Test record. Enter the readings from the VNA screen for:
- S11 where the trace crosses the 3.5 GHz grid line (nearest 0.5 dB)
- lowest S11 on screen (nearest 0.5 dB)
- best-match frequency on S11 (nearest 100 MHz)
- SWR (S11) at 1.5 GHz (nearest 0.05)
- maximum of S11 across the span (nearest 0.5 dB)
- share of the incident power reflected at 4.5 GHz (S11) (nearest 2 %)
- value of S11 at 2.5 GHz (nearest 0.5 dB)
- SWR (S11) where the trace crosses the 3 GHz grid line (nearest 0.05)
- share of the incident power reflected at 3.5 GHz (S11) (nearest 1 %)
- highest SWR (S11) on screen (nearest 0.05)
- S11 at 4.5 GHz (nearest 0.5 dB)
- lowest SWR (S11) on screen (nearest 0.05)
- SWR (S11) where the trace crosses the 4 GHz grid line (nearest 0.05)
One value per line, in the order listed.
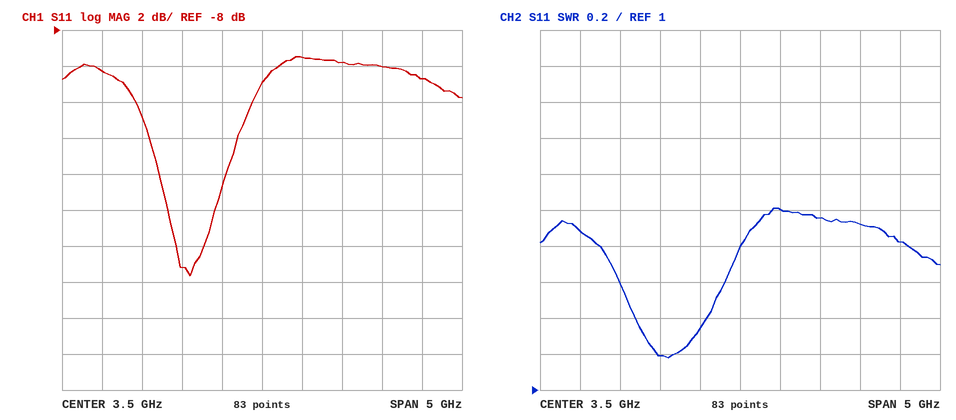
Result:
-11.0 dB
-21.5 dB
2.6 GHz
1.90
-9.5 dB
10 %
-21.0 dB
1.35
8 %
2.00
-10.0 dB
1.20
2.00
